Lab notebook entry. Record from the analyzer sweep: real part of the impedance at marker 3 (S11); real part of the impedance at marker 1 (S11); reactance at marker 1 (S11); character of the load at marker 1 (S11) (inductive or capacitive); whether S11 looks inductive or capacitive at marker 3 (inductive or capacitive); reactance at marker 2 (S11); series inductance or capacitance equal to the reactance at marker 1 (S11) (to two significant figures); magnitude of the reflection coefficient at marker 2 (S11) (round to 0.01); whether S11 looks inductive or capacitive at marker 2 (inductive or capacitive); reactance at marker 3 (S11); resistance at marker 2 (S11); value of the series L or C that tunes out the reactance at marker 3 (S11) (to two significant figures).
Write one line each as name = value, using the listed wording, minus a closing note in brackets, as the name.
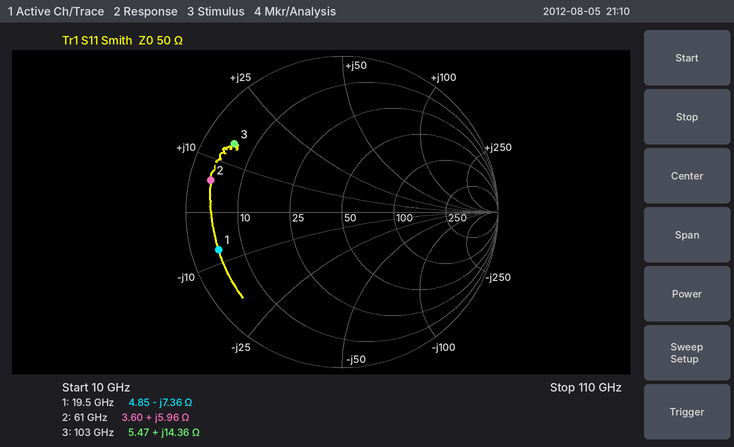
real part of the impedance at marker 3 = 5.47 Ω
real part of the impedance at marker 1 = 4.85 Ω
reactance at marker 1 = -7.36 Ω
character of the load at marker 1 (S11) = capacitive
whether S11 looks inductive or capacitive at marker 3 = inductive
reactance at marker 2 = +5.96 Ω
series inductance or capacitance equal to the reactance at marker 1 (S11) = 1.1 pF
magnitude of the reflection coefficient at marker 2 (S11) = 0.87
whether S11 looks inductive or capacitive at marker 2 = inductive
reactance at marker 3 = +14.36 Ω
resistance at marker 2 = 3.60 Ω
value of the series L or C that tunes out the reactance at marker 3 (S11) = 110 fF
